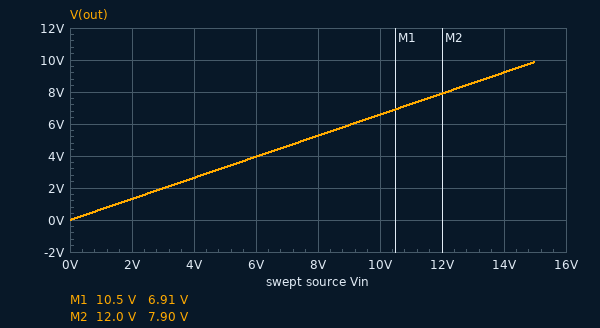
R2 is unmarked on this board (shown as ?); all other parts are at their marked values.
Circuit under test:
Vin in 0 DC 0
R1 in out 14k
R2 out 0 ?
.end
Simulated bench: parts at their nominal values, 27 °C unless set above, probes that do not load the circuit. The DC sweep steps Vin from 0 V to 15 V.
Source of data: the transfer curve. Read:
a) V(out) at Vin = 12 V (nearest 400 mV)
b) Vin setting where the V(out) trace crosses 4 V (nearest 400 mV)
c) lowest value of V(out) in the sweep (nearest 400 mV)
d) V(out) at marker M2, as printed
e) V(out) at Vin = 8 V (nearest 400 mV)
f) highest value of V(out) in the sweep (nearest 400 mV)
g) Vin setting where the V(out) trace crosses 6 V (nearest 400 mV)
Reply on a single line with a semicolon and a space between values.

8.0 V; 6.0 V; 0 V; 7.90 V; 5.2 V; 10.0 V; 9.2 V
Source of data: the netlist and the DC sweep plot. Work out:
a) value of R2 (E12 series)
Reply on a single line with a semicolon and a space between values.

27 kΩ
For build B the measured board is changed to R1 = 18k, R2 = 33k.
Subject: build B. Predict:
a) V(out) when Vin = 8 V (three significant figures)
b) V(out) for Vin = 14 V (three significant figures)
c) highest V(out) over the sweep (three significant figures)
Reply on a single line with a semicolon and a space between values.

5.18 V; 9.06 V; 9.71 V
